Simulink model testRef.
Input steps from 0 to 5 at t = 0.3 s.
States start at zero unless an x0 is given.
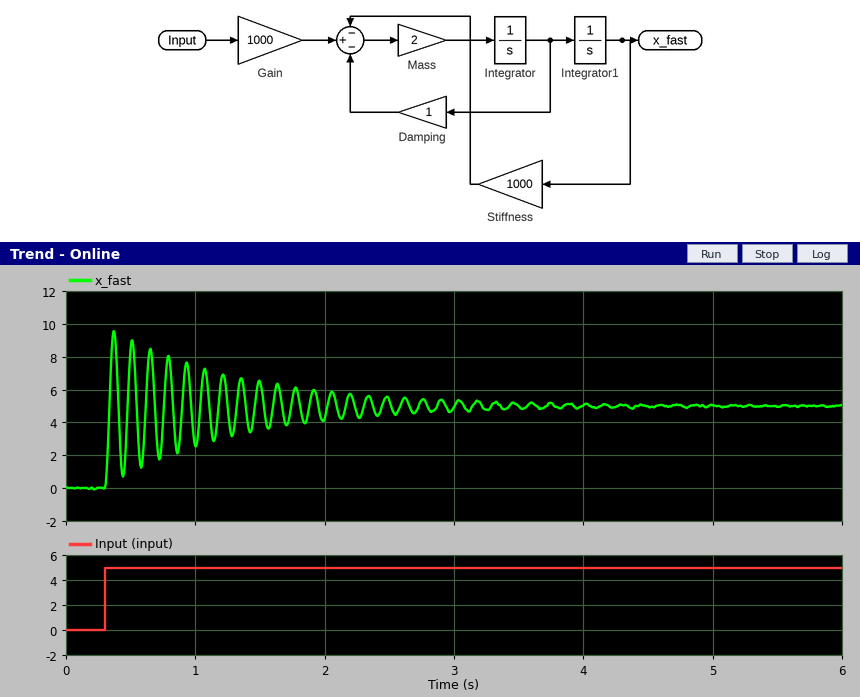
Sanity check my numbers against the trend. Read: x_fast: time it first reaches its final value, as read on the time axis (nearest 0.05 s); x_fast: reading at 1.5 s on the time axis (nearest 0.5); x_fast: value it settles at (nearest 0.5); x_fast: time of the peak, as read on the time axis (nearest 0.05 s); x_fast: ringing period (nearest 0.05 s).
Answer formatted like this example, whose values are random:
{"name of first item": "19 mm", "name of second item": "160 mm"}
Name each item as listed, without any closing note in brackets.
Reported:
{"x_fast: time it first reaches its final value, as read on the time axis": "0.35 s", "x_fast: reading at 1.5 s on the time axis": "6.5", "x_fast: value it settles at": "5.0", "x_fast: time of the peak, as read on the time axis": "0.35 s", "x_fast: ringing period": "0.15 s"}
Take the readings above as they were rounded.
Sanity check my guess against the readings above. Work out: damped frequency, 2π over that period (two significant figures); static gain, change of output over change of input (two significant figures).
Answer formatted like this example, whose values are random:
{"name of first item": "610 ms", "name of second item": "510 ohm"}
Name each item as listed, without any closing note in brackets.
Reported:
{"damped frequency, 2π over that period": "42 rad/s", "static gain, change of output over change of input": "1.0"}
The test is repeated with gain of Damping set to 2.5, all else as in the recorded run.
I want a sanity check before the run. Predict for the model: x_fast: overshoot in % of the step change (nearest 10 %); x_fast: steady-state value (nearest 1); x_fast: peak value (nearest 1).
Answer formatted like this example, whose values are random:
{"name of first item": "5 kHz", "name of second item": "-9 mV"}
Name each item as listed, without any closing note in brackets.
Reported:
{"x_fast: overshoot in % of the step change": "80 %", "x_fast: steady-state value": "5", "x_fast: peak value": "9"}
